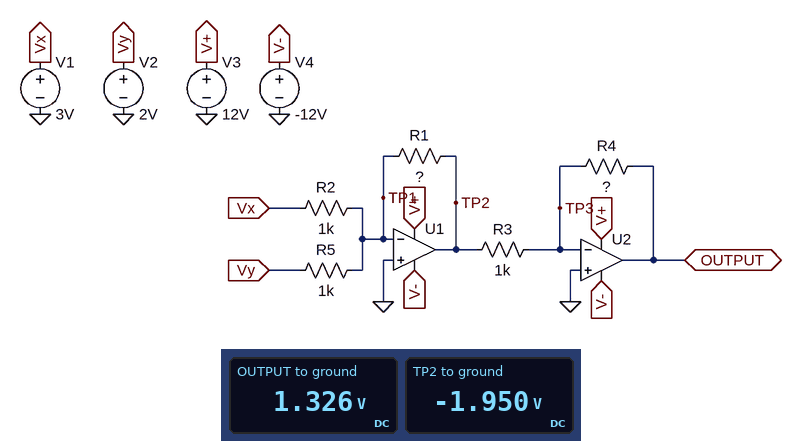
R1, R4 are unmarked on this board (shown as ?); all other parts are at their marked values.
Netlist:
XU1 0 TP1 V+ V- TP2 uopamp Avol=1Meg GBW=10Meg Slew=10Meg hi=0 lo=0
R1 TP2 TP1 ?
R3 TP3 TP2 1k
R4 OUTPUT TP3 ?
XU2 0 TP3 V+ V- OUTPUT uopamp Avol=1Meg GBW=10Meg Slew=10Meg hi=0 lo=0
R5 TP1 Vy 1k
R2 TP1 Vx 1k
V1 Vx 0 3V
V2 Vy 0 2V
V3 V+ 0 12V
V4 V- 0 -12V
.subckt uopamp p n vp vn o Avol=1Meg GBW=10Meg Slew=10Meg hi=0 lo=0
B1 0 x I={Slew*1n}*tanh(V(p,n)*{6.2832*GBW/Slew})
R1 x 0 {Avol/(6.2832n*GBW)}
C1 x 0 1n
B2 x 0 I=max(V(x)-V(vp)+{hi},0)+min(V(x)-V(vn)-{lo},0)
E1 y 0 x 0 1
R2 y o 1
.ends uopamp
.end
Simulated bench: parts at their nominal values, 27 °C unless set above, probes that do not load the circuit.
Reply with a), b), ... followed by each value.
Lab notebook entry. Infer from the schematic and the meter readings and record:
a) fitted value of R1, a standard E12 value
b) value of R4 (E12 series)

a) 390 Ω
b) 680 Ω
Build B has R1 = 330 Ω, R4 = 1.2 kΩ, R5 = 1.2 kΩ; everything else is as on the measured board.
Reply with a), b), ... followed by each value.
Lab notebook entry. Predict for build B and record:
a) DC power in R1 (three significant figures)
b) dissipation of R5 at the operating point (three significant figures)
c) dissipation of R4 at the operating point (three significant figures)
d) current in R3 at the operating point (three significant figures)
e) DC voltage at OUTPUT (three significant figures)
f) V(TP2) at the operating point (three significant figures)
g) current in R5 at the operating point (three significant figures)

a) 7.19 mW
b) 3.33 mW
c) 2.85 mW
d) 1.54 mA
e) 1.85 V
f) -1.54 V
g) 1.67 mA
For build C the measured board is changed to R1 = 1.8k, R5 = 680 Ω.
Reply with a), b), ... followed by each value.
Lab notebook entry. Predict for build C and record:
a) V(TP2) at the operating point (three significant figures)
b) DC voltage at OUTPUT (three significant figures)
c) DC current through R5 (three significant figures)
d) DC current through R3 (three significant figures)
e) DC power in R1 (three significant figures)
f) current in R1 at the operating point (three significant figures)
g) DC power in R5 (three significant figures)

a) -10.7 V
b) 7.27 V
c) 2.94 mA
d) 10.7 mA
e) 63.5 mW
f) 5.94 mA
g) 5.88 mW
